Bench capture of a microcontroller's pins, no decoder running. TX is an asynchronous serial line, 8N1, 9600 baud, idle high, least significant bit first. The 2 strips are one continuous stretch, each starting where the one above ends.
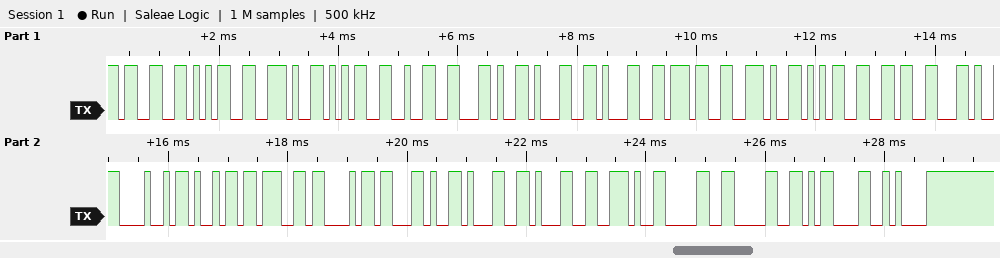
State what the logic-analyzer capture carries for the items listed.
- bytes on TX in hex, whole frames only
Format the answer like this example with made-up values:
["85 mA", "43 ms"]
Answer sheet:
["0x33 0x35 0x2E 0x35 0x32 0x2C 0x31 0x31 0x37 0x2E 0x35 0x36 0x2C 0x48 0x69 0x67 0x68 0x2C 0x31 0x31 0x2E 0x30 0x30 0x0D 0x0A"]
